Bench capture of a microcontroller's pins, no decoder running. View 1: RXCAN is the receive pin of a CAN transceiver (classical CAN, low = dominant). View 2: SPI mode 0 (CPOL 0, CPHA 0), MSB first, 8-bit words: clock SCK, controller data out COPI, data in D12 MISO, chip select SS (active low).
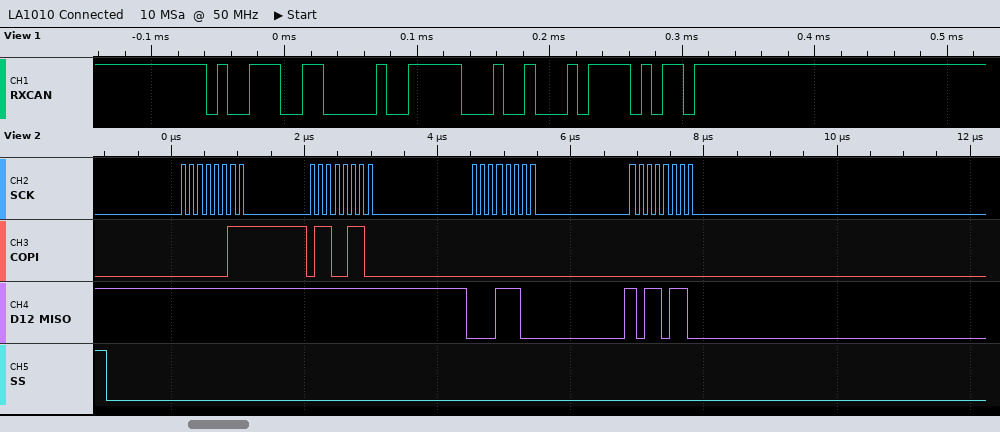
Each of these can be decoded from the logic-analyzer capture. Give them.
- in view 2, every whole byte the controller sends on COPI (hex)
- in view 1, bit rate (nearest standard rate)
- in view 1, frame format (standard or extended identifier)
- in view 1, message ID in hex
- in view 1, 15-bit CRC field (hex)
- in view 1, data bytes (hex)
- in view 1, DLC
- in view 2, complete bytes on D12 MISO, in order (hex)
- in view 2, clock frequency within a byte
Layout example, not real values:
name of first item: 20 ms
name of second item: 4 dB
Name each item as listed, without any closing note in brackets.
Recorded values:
in view 2, every whole byte the controller sends on COPI: 0x03 0x66 0x00 0x00
in view 1, bit rate: 125 kbit/s
in view 1, frame format: standard
in view 1, message ID in hex: 0x4E6
in view 1, 15-bit CRC field: 0x22F5
in view 1, data bytes: F2
in view 1, DLC: 1
in view 2, complete bytes on D12 MISO, in order: 0xFF 0xFF 0x1C 0xB6
in view 2, clock frequency within a byte: 8 MHz
